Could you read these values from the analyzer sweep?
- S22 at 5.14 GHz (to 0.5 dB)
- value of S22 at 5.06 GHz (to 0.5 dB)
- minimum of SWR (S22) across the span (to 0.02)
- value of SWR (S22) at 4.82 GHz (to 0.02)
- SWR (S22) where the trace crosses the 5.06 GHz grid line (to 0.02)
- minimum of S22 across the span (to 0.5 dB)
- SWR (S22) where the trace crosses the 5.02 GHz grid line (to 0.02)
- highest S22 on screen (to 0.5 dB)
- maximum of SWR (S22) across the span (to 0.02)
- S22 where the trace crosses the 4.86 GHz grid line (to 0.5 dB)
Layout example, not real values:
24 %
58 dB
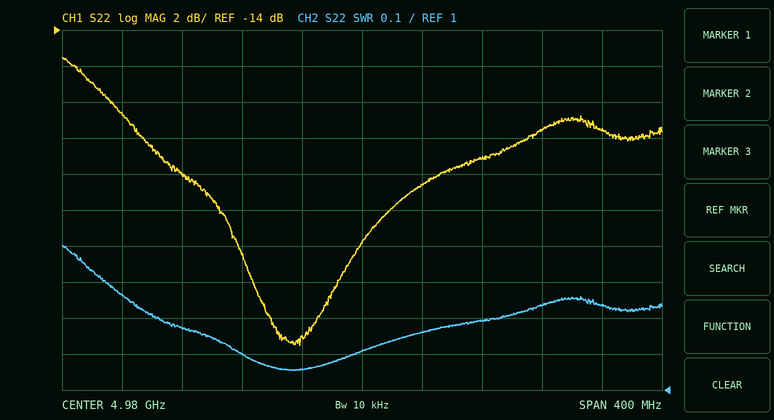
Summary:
-19.5 dB
-21.0 dB
1.06
1.26
1.20
-31.5 dB
1.16
-15.5 dB
1.40
-22.0 dB
